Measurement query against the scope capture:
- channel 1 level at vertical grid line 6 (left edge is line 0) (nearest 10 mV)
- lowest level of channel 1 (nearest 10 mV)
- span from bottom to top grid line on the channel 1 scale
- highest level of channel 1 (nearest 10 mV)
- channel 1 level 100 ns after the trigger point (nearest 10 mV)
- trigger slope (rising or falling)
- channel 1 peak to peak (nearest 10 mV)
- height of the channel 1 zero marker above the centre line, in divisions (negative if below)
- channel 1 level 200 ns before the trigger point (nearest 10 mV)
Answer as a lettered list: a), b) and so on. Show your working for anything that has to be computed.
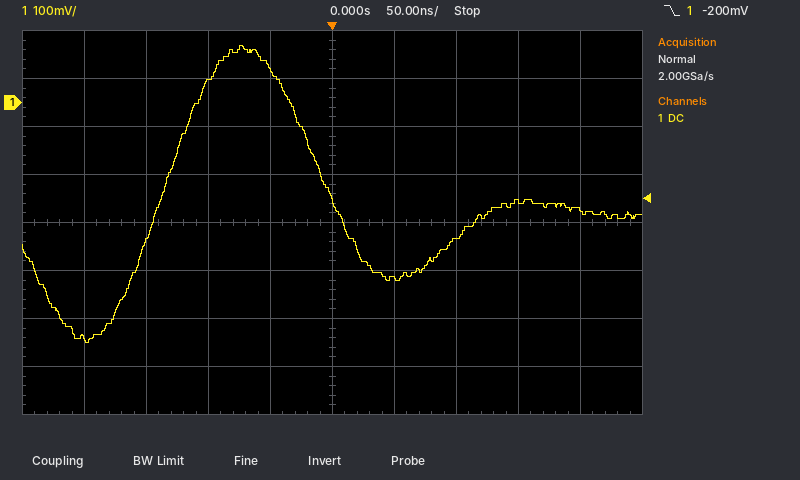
a) -370 mV
b) -500 mV
c) 800 mV
d) 120 mV
e) -280 mV
f) falling
g) 120 mV − (-500 mV) = 620 mV
h) +2.5 div
i) -490 mV
